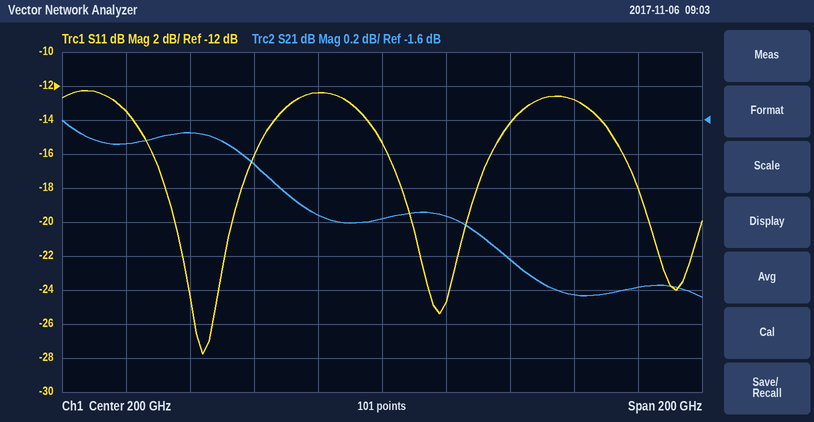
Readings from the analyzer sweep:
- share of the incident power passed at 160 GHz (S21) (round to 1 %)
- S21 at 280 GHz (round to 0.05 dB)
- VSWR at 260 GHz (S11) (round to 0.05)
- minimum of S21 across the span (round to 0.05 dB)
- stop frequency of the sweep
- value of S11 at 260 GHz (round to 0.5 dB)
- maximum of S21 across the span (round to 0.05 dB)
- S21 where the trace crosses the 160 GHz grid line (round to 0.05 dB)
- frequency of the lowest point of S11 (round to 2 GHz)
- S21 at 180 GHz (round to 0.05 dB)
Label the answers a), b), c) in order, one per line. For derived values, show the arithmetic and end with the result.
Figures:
a) 10^(-1.85/10) ≈ 65 %
b) -2.60 dB
c) |Γ| = 10^(-13/20) = 0.2239; VSWR = (1 + 0.2239)/(1 − 0.2239) ≈ 1.58, so 1.60 to the nearest 0.05
d) -2.65 dB
e) 300 GHz
f) -13.0 dB
g) -1.60 dB
h) -1.85 dB
i) 144 GHz
j) -2.15 dB
